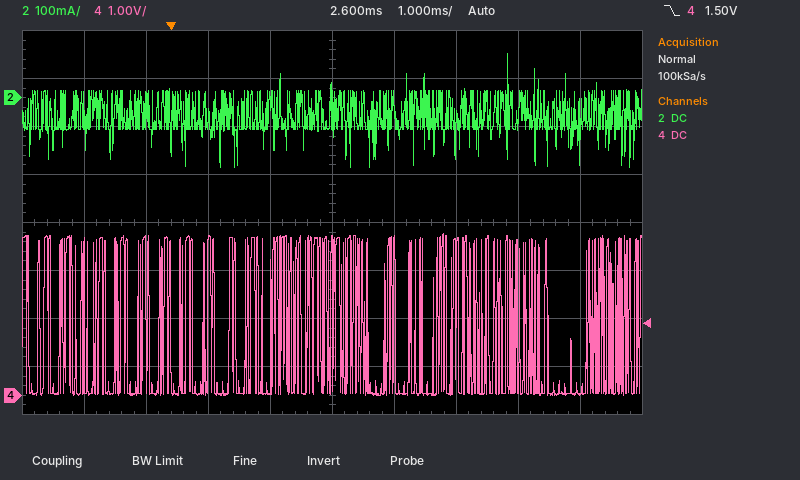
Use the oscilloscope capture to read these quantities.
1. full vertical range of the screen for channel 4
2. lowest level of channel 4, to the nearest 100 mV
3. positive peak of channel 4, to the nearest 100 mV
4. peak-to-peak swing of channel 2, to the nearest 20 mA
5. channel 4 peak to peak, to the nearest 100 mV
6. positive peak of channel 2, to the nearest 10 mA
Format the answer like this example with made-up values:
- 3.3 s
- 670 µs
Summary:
- 8 V
- 0.0 V
- 3.4 V
- 240 mA
- 3.4 V
- 90 mA
